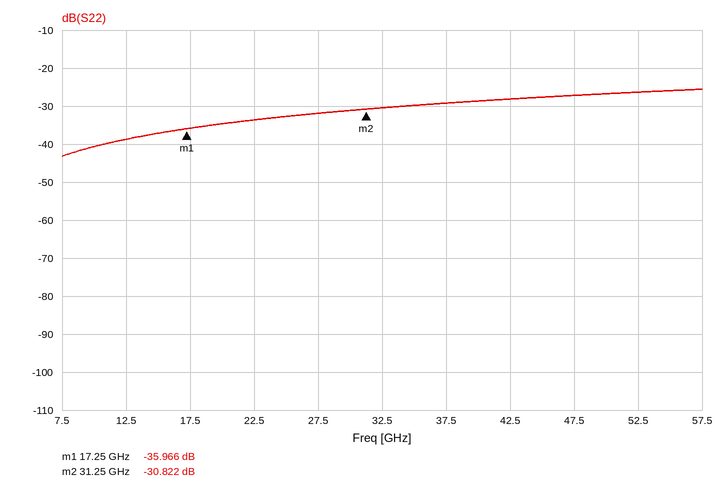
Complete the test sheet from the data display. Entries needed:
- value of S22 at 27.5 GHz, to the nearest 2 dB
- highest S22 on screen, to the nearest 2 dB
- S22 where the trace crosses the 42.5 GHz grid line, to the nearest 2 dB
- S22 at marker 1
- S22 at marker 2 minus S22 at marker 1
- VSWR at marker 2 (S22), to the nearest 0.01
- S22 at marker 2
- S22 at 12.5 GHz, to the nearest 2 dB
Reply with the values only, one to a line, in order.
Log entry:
-32 dB
-26 dB
-28 dB
-35.966 dB
5.144 dB
1.06
-30.822 dB
-38 dB
